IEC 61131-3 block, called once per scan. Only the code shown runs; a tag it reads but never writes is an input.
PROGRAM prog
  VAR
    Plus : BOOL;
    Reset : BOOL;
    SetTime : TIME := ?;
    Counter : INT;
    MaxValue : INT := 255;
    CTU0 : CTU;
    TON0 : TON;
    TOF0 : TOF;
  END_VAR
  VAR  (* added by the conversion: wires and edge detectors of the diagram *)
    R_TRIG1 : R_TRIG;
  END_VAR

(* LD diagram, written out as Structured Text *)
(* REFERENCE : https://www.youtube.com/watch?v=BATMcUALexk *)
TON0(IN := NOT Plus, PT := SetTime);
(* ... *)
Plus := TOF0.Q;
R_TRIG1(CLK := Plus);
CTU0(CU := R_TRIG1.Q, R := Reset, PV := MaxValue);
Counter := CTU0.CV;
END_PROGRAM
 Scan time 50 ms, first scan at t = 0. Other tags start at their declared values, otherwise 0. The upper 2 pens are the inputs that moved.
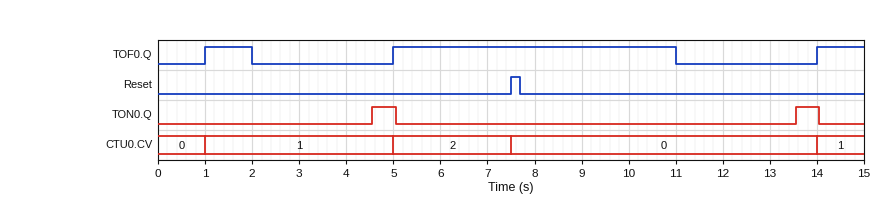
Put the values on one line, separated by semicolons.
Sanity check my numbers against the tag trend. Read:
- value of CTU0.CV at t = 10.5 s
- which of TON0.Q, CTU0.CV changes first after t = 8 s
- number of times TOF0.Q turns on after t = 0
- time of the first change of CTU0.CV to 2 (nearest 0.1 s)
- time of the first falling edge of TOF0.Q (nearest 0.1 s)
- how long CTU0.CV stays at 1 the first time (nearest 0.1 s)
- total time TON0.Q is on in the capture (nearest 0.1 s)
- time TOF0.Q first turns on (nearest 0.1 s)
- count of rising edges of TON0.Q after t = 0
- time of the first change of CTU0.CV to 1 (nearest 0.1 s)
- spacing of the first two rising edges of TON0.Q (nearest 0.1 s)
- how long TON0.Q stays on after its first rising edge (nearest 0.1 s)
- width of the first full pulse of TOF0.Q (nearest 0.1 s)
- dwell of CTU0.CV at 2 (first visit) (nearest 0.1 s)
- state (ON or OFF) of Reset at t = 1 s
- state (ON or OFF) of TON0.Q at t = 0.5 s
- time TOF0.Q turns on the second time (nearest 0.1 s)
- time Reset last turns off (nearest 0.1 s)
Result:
0; TON0.Q; 3; 5.0 s; 2.0 s; 4.0 s; 1.0 s; 1.0 s; 2; 1.0 s; 9.0 s; 0.5 s; 1.0 s; 2.5 s; OFF; OFF; 5.0 s; 7.7 s
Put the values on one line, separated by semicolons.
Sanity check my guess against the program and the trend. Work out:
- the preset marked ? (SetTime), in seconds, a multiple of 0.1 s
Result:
2.5 s
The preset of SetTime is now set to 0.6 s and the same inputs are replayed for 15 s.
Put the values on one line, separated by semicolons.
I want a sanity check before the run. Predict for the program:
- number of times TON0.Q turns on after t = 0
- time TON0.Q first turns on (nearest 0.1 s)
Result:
3; 0.6 s
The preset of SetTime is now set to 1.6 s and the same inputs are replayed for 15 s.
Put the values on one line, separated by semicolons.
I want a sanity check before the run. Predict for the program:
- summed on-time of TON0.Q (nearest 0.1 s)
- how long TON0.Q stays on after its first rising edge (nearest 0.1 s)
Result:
2.8 s; 1.4 s
